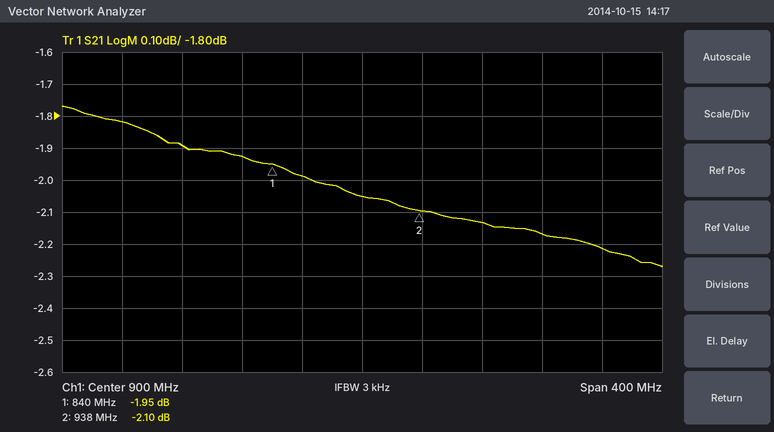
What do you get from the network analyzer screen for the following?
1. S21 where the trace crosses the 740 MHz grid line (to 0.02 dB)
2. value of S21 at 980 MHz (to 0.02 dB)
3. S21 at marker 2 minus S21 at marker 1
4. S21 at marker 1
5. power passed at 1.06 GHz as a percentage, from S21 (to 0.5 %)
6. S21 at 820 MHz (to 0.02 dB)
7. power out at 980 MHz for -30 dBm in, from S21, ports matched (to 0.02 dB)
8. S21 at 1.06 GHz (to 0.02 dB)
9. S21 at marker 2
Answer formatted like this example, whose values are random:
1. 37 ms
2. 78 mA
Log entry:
1. -1.82 dB
2. -2.14 dB
3. -0.15 dB
4. -1.95 dB
5. 60.0 %
6. -1.92 dB
7. -32.14 dBm
8. -2.22 dB
9. -2.10 dB
